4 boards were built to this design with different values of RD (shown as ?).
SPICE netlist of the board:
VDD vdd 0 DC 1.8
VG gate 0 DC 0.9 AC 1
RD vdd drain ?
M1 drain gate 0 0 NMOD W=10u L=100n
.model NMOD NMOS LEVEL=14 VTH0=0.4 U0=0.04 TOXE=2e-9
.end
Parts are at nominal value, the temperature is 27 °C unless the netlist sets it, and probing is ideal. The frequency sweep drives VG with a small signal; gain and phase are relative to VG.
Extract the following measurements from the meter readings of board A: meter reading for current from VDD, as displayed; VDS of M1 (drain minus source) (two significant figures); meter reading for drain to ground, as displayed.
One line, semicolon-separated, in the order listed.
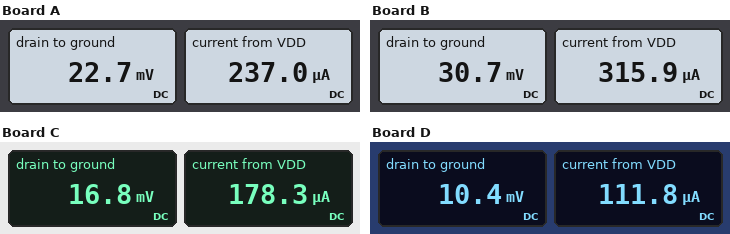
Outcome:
237.0 µA; 23 mV; 22.7 mV
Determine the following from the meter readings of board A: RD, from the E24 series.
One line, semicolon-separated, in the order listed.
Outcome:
7.5 kΩ
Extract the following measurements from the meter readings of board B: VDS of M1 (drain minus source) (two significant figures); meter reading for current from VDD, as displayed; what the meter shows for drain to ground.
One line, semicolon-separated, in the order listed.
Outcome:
31 mV; 315.9 µA; 30.7 mV
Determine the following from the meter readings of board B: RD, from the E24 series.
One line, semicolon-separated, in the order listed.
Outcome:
5.6 kΩ
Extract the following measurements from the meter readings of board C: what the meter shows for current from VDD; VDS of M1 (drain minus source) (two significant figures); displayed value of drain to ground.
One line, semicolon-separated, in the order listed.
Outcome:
178.3 µA; 17 mV; 16.8 mV
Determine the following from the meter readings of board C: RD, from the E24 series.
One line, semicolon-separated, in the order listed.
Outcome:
10 kΩ
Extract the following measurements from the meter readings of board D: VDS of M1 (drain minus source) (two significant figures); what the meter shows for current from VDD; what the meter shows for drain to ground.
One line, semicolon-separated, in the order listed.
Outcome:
10 mV; 111.8 µA; 10.4 mV
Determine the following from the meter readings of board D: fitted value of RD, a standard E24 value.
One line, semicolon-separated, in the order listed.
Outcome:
16 kΩ
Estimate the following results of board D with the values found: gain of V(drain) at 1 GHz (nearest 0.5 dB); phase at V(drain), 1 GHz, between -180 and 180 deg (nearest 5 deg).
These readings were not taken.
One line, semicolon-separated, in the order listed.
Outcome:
-31.5 dB; 145 deg
